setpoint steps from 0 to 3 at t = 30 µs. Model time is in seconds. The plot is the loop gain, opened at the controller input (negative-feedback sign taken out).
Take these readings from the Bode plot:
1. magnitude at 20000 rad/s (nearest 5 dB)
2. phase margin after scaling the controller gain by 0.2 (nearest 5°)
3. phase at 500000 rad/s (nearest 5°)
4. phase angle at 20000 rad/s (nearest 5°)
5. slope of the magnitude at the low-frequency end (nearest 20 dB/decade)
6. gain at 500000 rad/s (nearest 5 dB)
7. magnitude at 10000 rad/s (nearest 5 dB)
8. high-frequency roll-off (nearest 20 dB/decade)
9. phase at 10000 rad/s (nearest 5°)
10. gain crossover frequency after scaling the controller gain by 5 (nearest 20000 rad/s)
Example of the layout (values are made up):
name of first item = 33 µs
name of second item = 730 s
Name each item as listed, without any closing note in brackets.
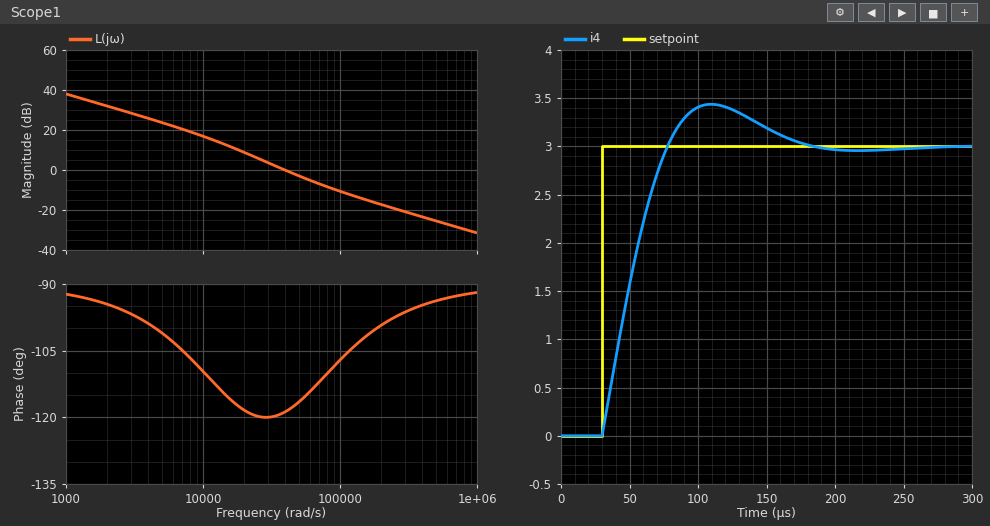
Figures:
magnitude at 20000 rad/s = 10 dB
phase margin after scaling the controller gain by 0.2 = 65°
phase at 500000 rad/s = -95°
phase angle at 20000 rad/s = -120°
slope of the magnitude at the low-frequency end = -20 dB/decade
gain at 500000 rad/s = -25 dB
magnitude at 10000 rad/s = 15 dB
high-frequency roll-off = -20 dB/decade
phase at 10000 rad/s = -110°
gain crossover frequency after scaling the controller gain by 5 = 140000 rad/s
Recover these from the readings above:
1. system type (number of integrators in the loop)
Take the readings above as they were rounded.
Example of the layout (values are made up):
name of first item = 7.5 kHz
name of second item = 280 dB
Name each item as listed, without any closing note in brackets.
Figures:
system type = 1
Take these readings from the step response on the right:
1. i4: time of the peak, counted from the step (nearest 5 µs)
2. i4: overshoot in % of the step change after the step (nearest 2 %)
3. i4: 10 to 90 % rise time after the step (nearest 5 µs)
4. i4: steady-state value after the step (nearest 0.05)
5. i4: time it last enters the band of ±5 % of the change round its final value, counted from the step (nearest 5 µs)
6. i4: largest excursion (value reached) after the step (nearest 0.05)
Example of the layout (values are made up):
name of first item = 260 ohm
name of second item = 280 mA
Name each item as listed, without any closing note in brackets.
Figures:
i4: time of the peak, counted from the step = 80 µs
i4: overshoot in % of the step change after the step = 14 %
i4: 10 to 90 % rise time after the step = 35 µs
i4: steady-state value after the step = 3.00
i4: time it last enters the band of ±5 % of the change round its final value, counted from the step = 125 µs
i4: largest excursion (value reached) after the step = 3.45
